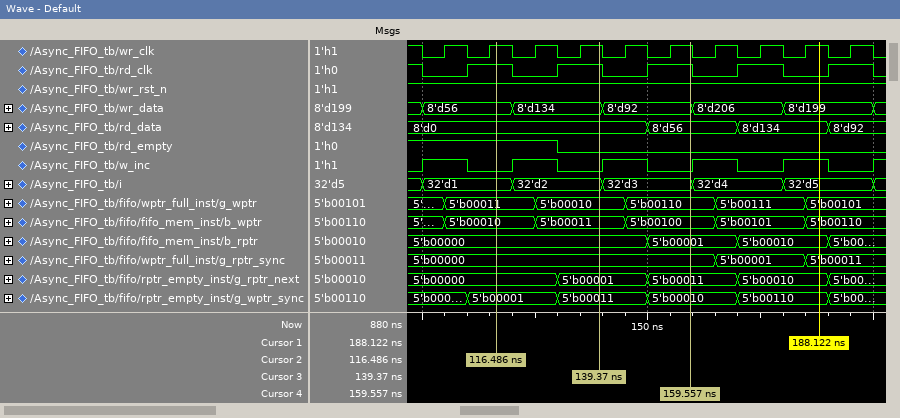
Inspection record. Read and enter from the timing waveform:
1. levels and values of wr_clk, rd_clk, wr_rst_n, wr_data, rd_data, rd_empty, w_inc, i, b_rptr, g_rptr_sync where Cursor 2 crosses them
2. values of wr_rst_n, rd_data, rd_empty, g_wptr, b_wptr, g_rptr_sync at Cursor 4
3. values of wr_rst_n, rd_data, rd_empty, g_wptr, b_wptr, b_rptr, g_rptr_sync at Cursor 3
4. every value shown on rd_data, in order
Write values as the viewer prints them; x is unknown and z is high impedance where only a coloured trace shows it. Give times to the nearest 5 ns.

wr_clk=1, rd_clk=1, wr_rst_n=1, wr_data=8'd56, rd_data=8'd0, rd_empty=1, w_inc=0, i=32'd1, b_rptr=5'b00000, g_rptr_sync=5'b00000
wr_rst_n=1, rd_data=8'd56, rd_empty=0, g_wptr=5'b00110, b_wptr=5'b00100, g_rptr_sync=5'b00000
wr_rst_n=1, rd_data=8'd0, rd_empty=0, g_wptr=5'b00010, b_wptr=5'b00011, b_rptr=5'b00000, g_rptr_sync=5'b00000
8'd0, 8'd56, 8'd134, 8'd92
